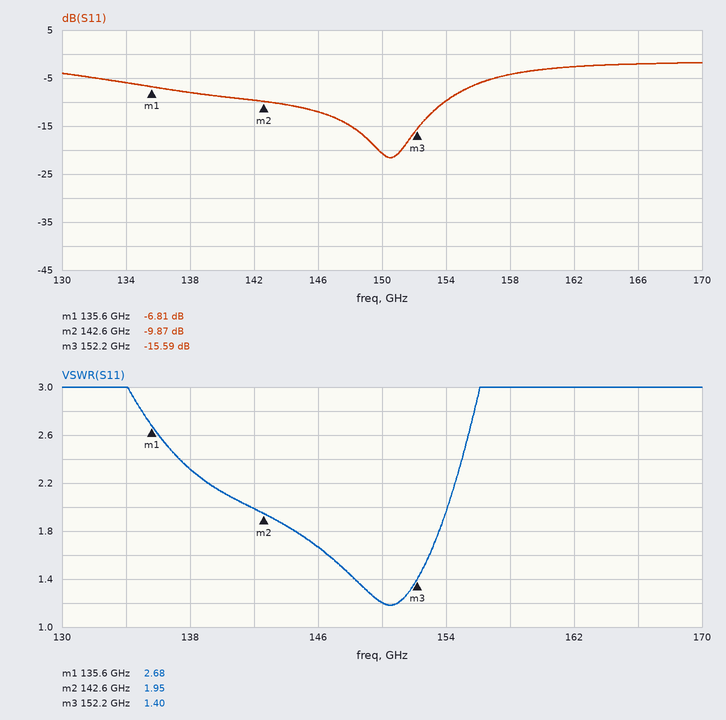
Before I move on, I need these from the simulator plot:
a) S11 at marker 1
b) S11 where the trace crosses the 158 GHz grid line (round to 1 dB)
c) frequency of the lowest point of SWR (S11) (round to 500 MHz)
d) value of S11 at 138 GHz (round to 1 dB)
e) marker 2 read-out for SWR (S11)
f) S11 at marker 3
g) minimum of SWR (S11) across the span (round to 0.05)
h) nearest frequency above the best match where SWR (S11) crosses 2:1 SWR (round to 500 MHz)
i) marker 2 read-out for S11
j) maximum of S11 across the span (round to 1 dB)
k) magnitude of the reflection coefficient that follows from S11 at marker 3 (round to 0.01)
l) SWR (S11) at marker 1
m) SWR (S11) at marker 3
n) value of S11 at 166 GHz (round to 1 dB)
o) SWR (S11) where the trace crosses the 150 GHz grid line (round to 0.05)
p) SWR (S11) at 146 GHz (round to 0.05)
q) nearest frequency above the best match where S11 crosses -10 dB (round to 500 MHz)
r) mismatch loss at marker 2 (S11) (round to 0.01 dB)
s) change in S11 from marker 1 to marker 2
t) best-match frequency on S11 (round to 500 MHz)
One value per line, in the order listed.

-6.81 dB
-4 dB
150.5 GHz
-8 dB
1.95
-15.59 dB
1.20
154.0 GHz
-9.87 dB
-2 dB
0.17
2.68
1.40
-2 dB
1.20
1.65
154.0 GHz
0.47 dB
-3.06 dB
150.5 GHz
